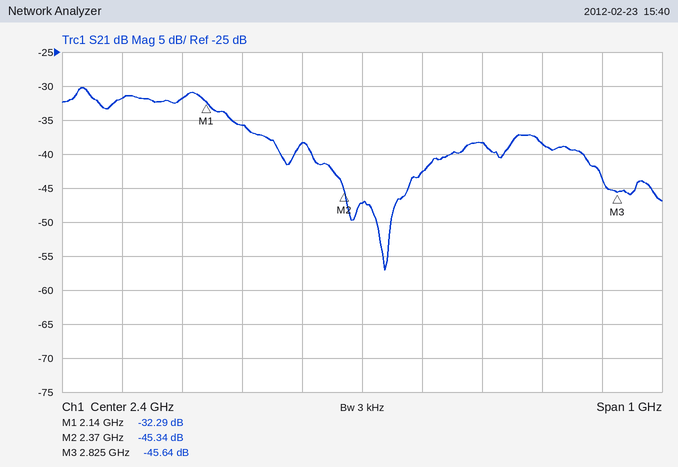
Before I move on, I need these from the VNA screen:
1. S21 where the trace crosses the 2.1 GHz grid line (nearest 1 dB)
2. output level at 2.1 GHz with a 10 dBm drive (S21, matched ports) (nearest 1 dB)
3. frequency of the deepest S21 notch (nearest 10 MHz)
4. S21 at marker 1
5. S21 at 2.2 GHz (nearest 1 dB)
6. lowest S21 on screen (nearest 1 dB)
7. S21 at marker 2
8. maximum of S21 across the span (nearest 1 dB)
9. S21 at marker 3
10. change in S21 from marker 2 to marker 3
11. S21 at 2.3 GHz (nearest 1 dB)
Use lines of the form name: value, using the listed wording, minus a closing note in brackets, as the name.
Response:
S21 where the trace crosses the 2.1 GHz grid line: -32 dB
output level at 2.1 GHz with a 10 dBm drive (S21, matched ports): -22 dBm
frequency of the deepest S21 notch: 2.44 GHz
S21 at marker 1: -32.29 dB
S21 at 2.2 GHz: -36 dB
lowest S21 on screen: -57 dB
S21 at marker 2: -45.34 dB
maximum of S21 across the span: -30 dB
S21 at marker 3: -45.64 dB
change in S21 from marker 2 to marker 3: -0.30 dB
S21 at 2.3 GHz: -38 dB
